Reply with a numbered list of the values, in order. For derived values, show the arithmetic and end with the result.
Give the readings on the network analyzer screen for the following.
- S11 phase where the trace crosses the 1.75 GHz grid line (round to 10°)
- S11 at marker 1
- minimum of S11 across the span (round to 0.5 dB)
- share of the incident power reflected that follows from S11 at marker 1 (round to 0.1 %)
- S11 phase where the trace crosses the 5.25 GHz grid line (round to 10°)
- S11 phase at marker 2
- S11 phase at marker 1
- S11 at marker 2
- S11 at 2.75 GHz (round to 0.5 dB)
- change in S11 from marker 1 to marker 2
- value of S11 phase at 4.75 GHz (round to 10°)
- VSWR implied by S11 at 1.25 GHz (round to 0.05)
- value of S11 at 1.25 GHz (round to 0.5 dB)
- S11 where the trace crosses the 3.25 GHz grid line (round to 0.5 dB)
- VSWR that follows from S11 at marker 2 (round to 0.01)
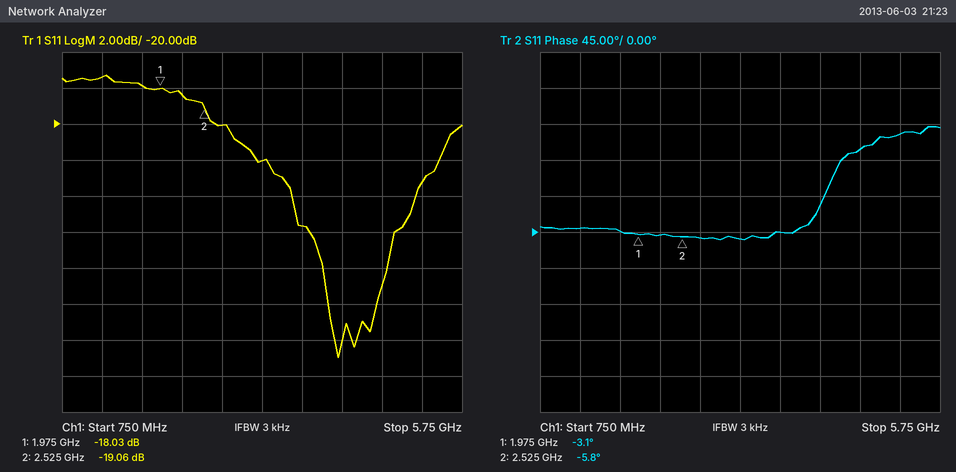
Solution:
1. 0°
2. -18.03 dB
3. -33.0 dB
4. 10^(-18.03/10) ≈ 1.6 %
5. 120°
6. -5.8°
7. -3.1°
8. -19.06 dB
9. -20.0 dB
10. -19.06 − (-18.03) = -1.03 dB
11. 100°
12. |Γ| = 10^(-17.5/20) = 0.1334; VSWR = (1 + 0.1334)/(1 − 0.1334) ≈ 1.31, so 1.30 to the nearest 0.05
13. -17.5 dB
14. -22.0 dB
15. (1 + 0.1114)/(1 − 0.1114) ≈ 1.25
